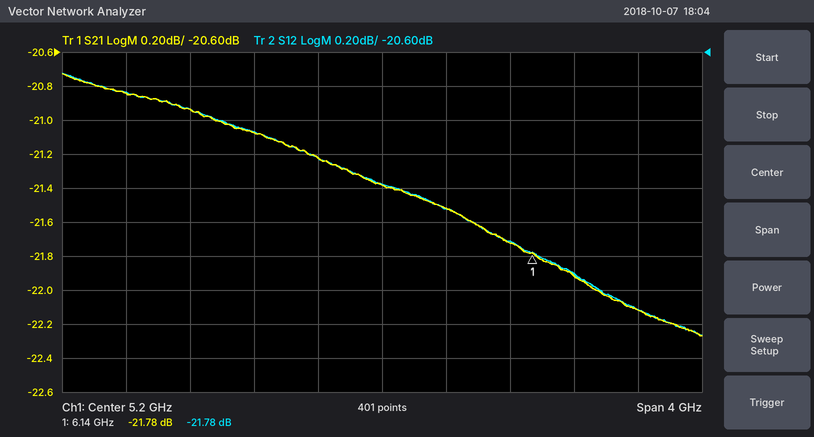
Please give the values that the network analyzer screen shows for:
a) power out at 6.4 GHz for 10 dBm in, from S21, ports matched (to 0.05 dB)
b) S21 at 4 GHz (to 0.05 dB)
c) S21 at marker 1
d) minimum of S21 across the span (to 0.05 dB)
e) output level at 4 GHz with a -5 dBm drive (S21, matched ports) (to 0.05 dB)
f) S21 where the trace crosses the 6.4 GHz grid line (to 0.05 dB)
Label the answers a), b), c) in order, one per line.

a) -11.90 dBm
b) -20.95 dB
c) -21.78 dB
d) -22.25 dB
e) -25.95 dBm
f) -21.90 dB
